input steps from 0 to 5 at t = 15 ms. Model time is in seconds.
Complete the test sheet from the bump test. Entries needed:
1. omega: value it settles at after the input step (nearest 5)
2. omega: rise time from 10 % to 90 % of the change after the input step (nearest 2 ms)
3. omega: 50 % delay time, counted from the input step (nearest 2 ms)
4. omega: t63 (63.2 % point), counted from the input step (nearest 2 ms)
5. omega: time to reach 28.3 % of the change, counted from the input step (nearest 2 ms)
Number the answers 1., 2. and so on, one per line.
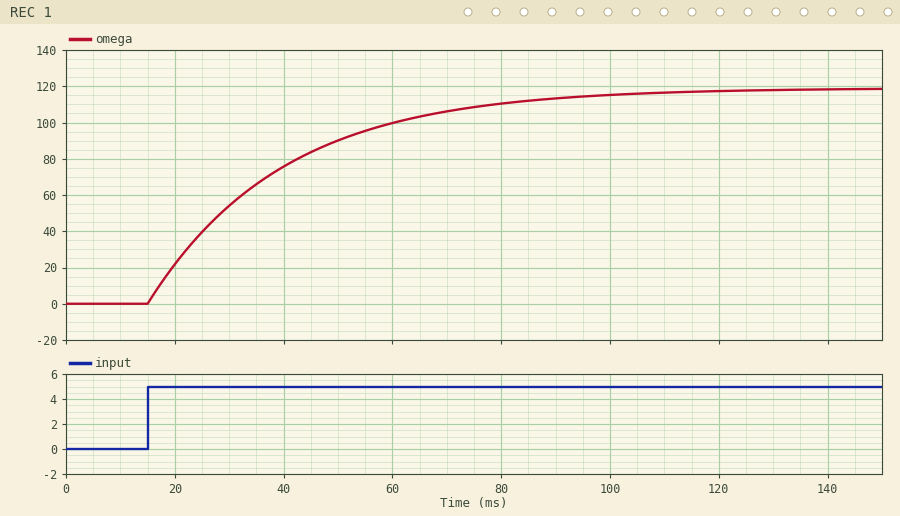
1. 120
2. 54 ms
3. 18 ms
4. 24 ms
5. 8 ms
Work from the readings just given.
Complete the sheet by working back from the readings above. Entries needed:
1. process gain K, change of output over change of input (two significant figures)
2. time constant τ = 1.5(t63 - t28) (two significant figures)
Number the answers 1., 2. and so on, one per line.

1. 24
2. 24 ms
